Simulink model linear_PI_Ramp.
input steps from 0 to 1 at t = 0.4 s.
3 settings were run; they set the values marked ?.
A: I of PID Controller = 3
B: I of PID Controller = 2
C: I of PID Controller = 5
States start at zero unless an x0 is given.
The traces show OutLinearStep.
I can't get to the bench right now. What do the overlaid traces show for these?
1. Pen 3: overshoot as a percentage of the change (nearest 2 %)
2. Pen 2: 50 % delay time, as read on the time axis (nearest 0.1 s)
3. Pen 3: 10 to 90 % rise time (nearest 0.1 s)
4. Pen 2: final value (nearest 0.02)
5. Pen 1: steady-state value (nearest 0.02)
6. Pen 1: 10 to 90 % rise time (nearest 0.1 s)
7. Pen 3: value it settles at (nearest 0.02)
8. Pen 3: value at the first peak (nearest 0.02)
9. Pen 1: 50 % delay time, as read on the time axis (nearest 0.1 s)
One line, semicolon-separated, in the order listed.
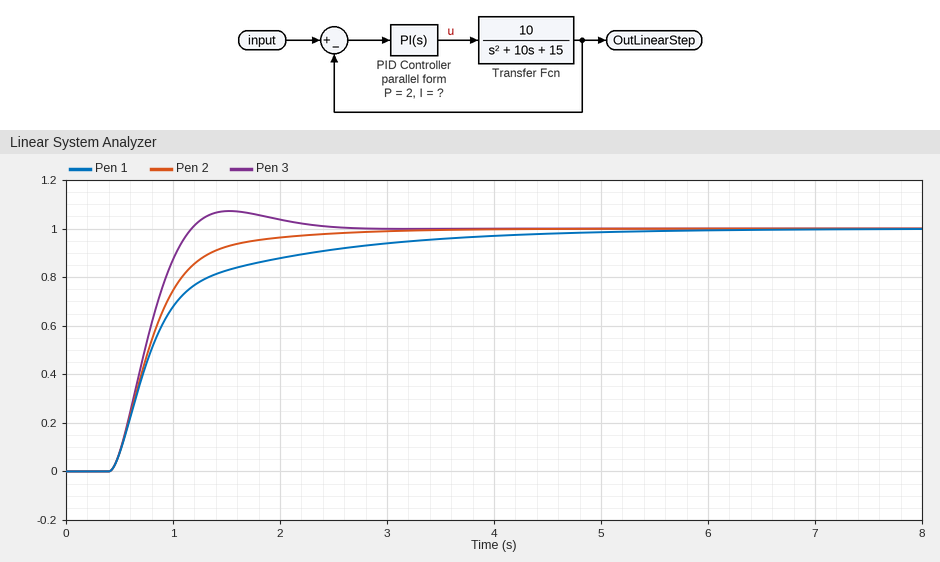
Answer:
8 %; 0.8 s; 0.5 s; 1.00; 1.00; 1.8 s; 1.00; 1.08; 0.8 s
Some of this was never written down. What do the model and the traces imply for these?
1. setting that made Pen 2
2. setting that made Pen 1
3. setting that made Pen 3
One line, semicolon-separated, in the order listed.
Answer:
A; B; C
